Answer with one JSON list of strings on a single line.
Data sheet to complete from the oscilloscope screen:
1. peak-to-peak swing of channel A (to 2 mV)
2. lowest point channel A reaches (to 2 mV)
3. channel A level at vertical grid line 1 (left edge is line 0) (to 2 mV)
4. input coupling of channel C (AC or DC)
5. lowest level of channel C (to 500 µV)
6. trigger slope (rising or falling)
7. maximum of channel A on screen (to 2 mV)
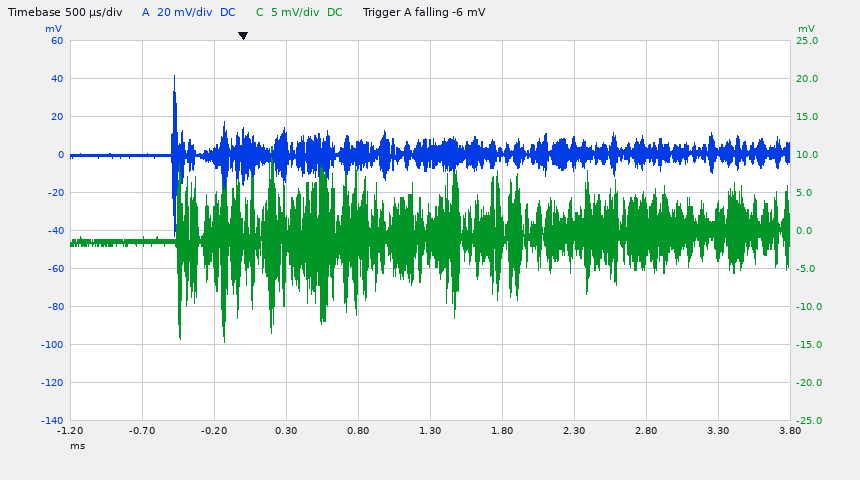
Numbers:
["84 mV", "-42 mV", "0 mV", "DC", "-14.5 mV", "falling", "42 mV"]
